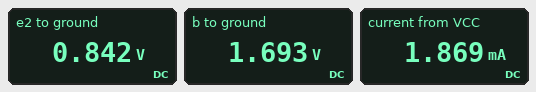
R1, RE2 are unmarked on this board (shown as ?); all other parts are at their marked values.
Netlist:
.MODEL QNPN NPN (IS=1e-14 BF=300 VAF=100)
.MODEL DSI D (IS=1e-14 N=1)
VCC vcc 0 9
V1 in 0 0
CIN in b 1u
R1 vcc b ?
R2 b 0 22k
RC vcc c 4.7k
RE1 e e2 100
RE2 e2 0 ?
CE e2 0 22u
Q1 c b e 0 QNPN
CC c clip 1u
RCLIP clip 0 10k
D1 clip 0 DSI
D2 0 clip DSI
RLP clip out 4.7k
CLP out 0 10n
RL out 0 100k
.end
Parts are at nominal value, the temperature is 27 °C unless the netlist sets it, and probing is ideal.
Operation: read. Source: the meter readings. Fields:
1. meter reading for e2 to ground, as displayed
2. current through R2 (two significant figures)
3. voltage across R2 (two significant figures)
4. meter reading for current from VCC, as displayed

0.842 V
77 µA
1.7 V
1.869 mA
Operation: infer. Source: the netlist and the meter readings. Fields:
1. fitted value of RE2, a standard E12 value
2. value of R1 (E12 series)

470 Ω
39 kΩ
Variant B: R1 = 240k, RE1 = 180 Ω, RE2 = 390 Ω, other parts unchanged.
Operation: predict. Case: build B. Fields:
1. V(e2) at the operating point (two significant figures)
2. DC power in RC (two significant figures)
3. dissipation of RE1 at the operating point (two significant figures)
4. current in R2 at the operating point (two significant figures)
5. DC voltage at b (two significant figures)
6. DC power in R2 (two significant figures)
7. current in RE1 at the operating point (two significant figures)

87 mV
230 µW
9.0 µW
34 µA
740 mV
25 µW
220 µA
